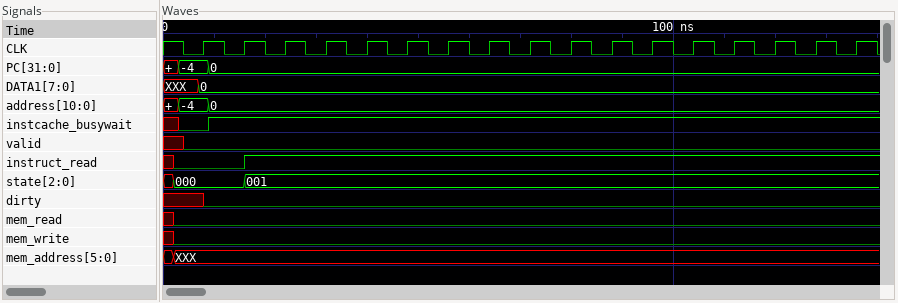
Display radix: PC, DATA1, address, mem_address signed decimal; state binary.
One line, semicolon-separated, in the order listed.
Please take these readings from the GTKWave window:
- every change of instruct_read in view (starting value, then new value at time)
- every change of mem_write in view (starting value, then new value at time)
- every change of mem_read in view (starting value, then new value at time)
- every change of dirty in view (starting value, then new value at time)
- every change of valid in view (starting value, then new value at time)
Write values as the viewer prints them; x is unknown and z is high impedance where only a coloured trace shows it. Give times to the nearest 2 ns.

x, 0 at 2 ns, 1 at 16 ns; x, 0 at 2 ns; x, 0 at 2 ns; x, 0 at 8 ns; x, 0 at 4 ns
